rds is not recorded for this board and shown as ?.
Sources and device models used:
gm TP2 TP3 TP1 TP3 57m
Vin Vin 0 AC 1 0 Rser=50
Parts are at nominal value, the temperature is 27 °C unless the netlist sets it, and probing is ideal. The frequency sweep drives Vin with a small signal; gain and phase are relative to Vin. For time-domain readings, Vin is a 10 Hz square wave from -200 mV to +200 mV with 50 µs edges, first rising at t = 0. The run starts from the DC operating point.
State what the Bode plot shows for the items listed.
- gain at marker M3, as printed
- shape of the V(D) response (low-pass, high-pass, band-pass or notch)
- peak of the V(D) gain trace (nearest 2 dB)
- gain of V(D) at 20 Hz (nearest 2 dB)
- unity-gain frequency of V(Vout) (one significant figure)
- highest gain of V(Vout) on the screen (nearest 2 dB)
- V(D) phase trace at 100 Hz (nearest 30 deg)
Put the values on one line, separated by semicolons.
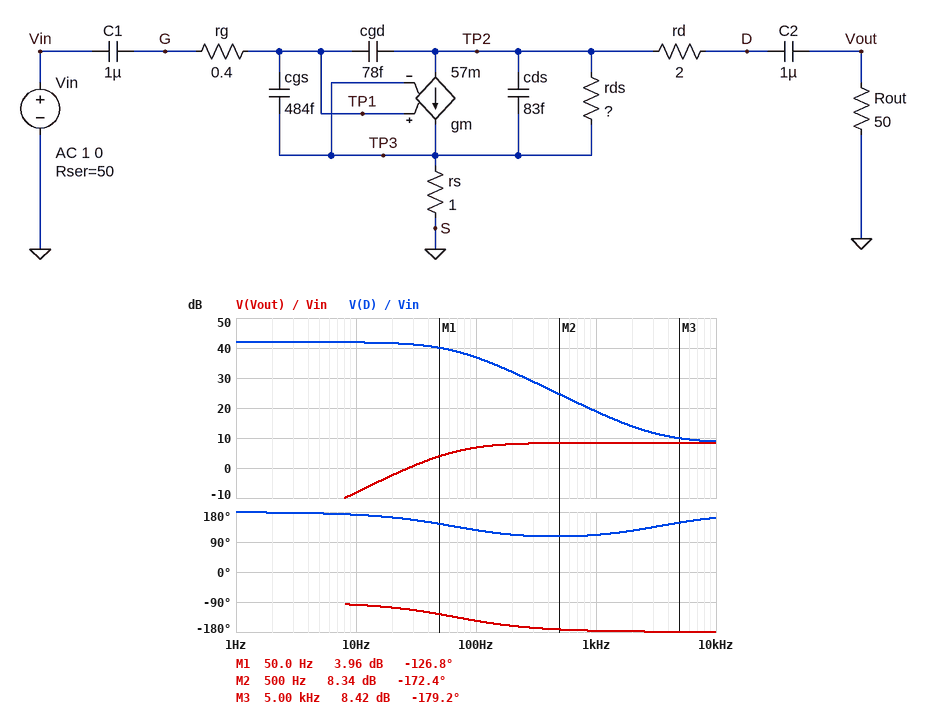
8.42 dB; low-pass; 42 dB; 42 dB; 30 Hz; 8 dB; 120 deg
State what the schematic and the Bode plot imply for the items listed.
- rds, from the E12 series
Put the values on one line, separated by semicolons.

2.2 kΩ
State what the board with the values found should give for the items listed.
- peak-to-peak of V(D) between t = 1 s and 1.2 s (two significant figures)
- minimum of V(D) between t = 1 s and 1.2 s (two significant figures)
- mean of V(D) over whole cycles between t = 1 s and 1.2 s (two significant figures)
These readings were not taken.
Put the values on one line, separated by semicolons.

50 V; -50 V; -25 V
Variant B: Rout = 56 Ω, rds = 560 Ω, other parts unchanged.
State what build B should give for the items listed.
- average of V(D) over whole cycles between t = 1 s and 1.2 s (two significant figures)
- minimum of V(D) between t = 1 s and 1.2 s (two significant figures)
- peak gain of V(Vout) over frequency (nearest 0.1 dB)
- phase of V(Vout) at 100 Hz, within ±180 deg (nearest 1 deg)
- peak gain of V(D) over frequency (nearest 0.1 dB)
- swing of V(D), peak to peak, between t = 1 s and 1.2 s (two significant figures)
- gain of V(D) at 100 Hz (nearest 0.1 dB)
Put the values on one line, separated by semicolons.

-6.4 V; -13 V; 8.8 dB; -112 deg; 30.1 dB; 13 V; 29.4 dB
